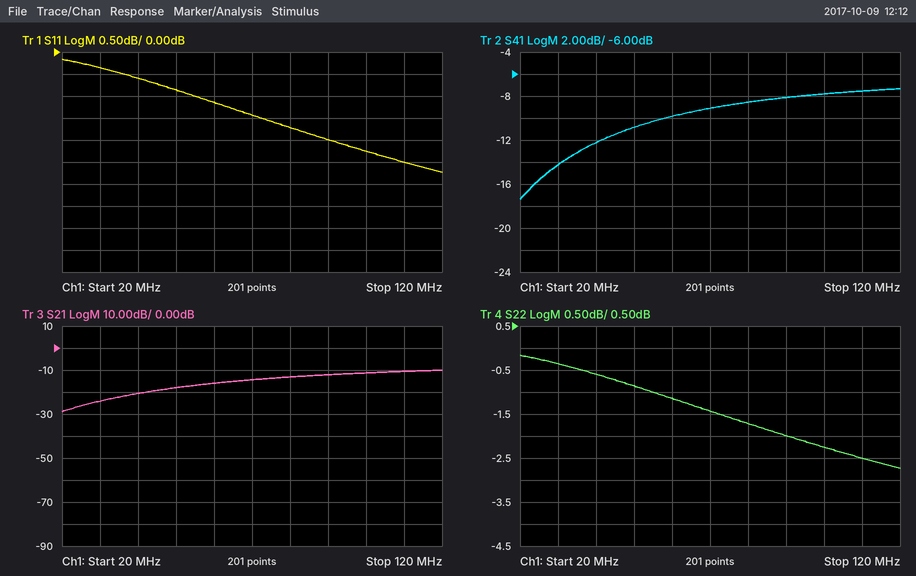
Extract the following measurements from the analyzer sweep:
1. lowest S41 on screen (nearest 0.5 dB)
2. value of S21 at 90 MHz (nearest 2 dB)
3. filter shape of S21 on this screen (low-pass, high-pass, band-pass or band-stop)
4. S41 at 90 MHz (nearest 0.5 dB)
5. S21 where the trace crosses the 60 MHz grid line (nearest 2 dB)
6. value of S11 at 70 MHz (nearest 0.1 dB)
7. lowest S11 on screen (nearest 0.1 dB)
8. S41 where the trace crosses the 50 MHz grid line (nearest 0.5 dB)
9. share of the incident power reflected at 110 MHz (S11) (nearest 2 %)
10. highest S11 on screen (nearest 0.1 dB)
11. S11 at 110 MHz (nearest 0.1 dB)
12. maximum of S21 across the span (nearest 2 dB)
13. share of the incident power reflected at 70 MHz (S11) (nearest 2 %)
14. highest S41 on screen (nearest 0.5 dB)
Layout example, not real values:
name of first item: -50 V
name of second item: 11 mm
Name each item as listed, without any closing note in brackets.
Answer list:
lowest S41 on screen: -17.5 dB
value of S21 at 90 MHz: -12 dB
filter shape of S21 on this screen: high-pass
S41 at 90 MHz: -8.0 dB
S21 where the trace crosses the 60 MHz grid line: -16 dB
value of S11 at 70 MHz: -1.4 dB
lowest S11 on screen: -2.7 dB
S41 where the trace crosses the 50 MHz grid line: -11.0 dB
share of the incident power reflected at 110 MHz (S11): 56 %
highest S11 on screen: -0.2 dB
S11 at 110 MHz: -2.5 dB
maximum of S21 across the span: -10 dB
share of the incident power reflected at 70 MHz (S11): 72 %
highest S41 on screen: -7.5 dB
